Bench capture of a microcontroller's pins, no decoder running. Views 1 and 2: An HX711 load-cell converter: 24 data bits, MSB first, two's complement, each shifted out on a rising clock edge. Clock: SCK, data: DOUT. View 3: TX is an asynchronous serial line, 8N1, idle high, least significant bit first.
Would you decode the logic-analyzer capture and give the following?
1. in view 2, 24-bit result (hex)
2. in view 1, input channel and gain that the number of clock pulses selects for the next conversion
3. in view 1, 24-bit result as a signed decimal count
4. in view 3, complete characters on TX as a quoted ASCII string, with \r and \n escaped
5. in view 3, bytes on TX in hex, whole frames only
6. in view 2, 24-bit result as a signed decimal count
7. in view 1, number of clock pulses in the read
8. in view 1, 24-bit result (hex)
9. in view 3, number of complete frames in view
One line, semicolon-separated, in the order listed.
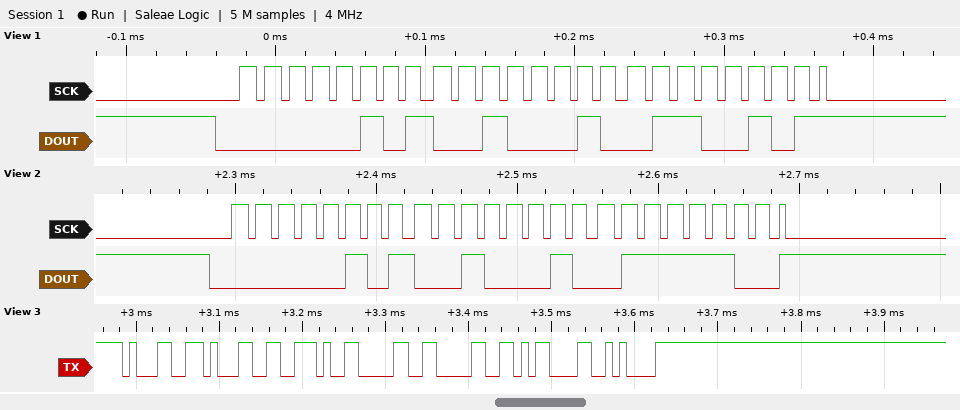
0x05227C; channel A, gain 128; 336485; "11.00\r\n"; 0x31 0x31 0x2E 0x30 0x30 0x0D 0x0A; 336508; 25; 0x052265; 7
